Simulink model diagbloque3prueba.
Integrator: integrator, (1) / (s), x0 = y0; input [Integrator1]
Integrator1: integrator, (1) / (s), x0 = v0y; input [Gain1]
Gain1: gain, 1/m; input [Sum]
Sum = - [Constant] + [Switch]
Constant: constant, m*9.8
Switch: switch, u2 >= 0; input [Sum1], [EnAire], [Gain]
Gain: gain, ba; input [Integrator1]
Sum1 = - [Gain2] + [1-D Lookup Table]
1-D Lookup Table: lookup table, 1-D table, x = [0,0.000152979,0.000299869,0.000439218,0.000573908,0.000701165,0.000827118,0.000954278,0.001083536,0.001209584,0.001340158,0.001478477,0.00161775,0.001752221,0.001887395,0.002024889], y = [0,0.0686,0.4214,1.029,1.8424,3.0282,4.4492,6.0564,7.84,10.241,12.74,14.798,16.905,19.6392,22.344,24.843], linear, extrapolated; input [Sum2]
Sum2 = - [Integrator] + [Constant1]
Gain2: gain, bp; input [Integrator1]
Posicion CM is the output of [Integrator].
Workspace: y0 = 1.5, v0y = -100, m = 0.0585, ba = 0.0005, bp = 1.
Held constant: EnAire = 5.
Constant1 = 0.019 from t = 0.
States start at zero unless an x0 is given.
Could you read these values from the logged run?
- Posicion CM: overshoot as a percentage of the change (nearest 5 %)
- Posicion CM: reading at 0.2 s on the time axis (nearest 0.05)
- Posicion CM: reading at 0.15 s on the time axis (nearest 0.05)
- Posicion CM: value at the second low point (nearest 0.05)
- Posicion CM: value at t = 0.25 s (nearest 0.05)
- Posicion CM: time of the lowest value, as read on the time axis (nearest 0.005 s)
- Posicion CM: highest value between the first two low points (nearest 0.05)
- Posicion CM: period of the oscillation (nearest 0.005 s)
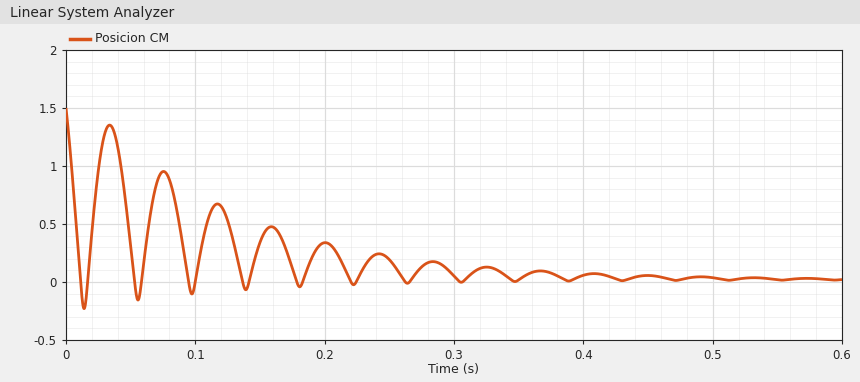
15 %
0.35
0.35
-0.15
0.20
0.015 s
1.35
0.040 s
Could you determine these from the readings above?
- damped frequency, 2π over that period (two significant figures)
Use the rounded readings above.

160 rad/s
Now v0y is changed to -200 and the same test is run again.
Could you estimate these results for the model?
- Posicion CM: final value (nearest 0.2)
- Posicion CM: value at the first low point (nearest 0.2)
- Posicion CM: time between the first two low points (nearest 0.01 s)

0.0
-0.4
0.04 s
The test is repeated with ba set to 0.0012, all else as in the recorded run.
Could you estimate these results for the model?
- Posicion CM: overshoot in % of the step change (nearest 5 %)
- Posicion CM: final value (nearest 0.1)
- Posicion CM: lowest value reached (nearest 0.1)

15 %
0.0
-0.2
